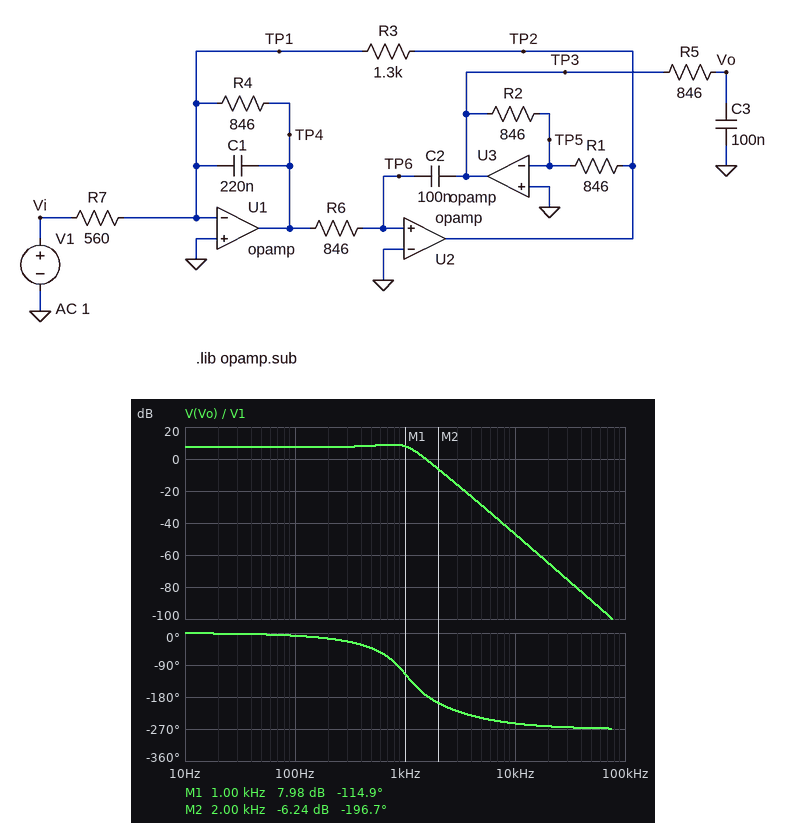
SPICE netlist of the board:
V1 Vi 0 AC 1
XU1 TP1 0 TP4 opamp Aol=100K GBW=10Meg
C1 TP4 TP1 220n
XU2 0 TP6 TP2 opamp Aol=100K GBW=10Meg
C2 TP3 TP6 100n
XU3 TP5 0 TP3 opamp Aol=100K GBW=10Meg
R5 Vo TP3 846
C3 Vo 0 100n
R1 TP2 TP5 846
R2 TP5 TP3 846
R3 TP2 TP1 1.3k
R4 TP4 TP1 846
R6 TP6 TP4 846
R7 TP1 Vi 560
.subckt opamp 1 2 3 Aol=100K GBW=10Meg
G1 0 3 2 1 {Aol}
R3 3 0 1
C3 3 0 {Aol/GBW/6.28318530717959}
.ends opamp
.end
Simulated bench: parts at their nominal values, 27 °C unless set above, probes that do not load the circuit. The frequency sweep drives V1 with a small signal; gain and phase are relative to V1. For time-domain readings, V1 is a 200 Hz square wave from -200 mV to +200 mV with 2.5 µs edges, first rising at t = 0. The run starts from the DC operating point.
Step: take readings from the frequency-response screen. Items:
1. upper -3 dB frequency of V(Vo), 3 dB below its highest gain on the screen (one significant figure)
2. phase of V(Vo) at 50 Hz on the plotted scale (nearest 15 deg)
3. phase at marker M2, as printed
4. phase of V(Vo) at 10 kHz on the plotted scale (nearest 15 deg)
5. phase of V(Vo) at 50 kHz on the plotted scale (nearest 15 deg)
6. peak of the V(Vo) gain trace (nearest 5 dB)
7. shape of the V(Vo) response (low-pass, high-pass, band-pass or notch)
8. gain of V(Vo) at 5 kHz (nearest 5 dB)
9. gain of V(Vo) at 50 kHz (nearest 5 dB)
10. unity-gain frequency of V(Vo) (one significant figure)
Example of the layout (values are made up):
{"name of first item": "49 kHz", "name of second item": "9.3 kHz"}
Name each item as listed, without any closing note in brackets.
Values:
{"upper -3 dB frequency of V(Vo), 3 dB below its highest gain on the screen": "1 kHz", "phase of V(Vo) at 50 Hz on the plotted scale": "0 deg", "phase at marker M2, as printed": "-196.7 deg", "phase of V(Vo) at 10 kHz on the plotted scale": "-255 deg", "phase of V(Vo) at 50 kHz on the plotted scale": "-270 deg", "peak of the V(Vo) gain trace": "10 dB", "shape of the V(Vo) response": "low-pass", "gain of V(Vo) at 5 kHz": "-30 dB", "gain of V(Vo) at 50 kHz": "-90 dB", "unity-gain frequency of V(Vo)": "2 kHz"}
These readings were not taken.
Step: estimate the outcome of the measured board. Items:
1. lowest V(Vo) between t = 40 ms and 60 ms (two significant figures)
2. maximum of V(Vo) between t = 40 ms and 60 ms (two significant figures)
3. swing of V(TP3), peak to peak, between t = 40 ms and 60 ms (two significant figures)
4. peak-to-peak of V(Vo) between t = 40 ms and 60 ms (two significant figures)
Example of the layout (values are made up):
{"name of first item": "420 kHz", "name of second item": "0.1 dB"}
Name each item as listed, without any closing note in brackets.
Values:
{"lowest V(Vo) between t = 40 ms and 60 ms": "-650 mV", "maximum of V(Vo) between t = 40 ms and 60 ms": "650 mV", "swing of V(TP3), peak to peak, between t = 40 ms and 60 ms": "1.4 V", "peak-to-peak of V(Vo) between t = 40 ms and 60 ms": "1.3 V"}
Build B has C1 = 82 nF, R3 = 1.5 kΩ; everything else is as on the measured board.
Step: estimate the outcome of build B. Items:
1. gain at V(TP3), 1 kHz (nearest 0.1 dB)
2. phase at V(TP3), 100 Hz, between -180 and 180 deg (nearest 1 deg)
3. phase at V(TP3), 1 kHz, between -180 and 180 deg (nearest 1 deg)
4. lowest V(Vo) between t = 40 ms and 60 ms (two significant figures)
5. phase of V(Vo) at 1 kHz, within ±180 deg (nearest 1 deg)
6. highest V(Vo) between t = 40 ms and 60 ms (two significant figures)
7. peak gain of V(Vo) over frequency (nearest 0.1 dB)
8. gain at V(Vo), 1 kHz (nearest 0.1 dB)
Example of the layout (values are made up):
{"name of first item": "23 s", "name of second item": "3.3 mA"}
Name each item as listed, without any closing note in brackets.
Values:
{"gain at V(TP3), 1 kHz": "7.6 dB", "phase at V(TP3), 100 Hz, between -180 and 180 deg": "-5 deg", "phase at V(TP3), 1 kHz, between -180 and 180 deg": "-58 deg", "lowest V(Vo) between t = 40 ms and 60 ms": "-550 mV", "phase of V(Vo) at 1 kHz, within ±180 deg": "-86 deg", "highest V(Vo) between t = 40 ms and 60 ms": "550 mV", "peak gain of V(Vo) over frequency": "8.6 dB", "gain at V(Vo), 1 kHz": "6.6 dB"}
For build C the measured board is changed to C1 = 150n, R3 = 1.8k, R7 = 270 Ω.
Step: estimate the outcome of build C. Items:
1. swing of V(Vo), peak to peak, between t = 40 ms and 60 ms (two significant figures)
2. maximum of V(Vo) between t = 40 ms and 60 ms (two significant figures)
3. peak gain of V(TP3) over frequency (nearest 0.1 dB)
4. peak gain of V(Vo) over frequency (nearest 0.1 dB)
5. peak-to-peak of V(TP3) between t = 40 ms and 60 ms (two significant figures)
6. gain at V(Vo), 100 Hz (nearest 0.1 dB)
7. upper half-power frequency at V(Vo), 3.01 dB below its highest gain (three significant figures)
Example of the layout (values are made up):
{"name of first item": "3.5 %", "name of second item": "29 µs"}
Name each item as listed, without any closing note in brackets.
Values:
{"swing of V(Vo), peak to peak, between t = 40 ms and 60 ms": "3.1 V", "maximum of V(Vo) between t = 40 ms and 60 ms": "1.5 V", "peak gain of V(TP3) over frequency": "16.9 dB", "peak gain of V(Vo) over frequency": "16.6 dB", "peak-to-peak of V(TP3) between t = 40 ms and 60 ms": "3.2 V", "gain at V(Vo), 100 Hz": "16.5 dB", "upper half-power frequency at V(Vo), 3.01 dB below its highest gain": "1.07 kHz"}
